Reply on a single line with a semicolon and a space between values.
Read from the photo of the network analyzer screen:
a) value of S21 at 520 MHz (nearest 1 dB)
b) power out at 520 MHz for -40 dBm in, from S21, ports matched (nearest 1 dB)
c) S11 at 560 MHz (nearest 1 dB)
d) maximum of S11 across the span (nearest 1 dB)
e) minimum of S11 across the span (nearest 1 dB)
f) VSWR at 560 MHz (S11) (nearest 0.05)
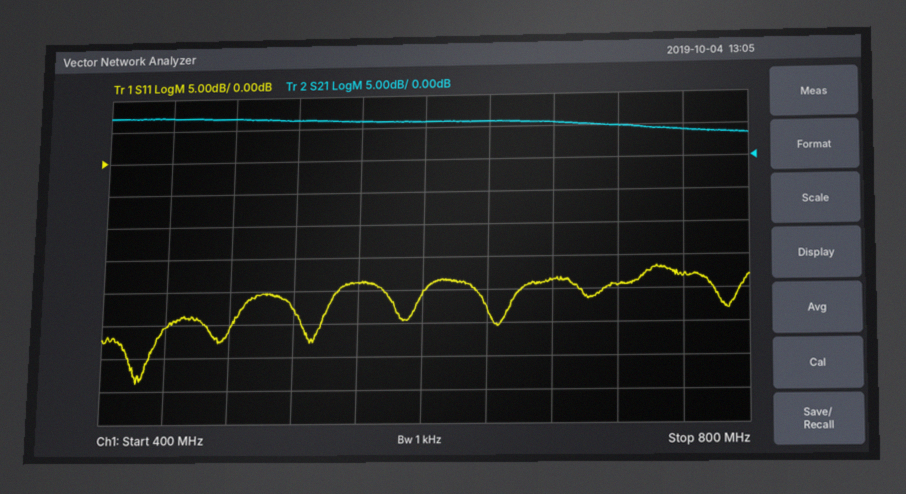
6 dB; -34 dBm; -19 dB; -17 dB; -34 dB; 1.25
